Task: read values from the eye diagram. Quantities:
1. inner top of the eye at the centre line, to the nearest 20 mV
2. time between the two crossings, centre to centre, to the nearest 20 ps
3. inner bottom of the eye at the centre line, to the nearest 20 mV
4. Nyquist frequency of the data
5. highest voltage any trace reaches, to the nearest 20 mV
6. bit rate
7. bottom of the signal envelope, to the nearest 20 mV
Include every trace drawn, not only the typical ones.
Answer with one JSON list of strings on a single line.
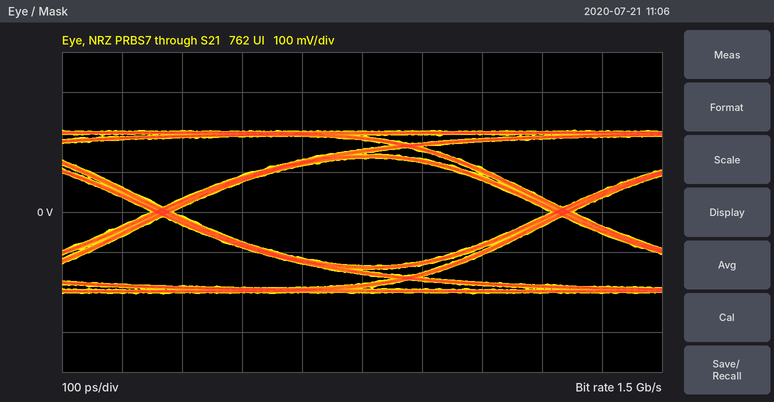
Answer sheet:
["140 mV", "660 ps", "-140 mV", "750 MHz", "200 mV", "1.5 Gb/s", "-200 mV"]
